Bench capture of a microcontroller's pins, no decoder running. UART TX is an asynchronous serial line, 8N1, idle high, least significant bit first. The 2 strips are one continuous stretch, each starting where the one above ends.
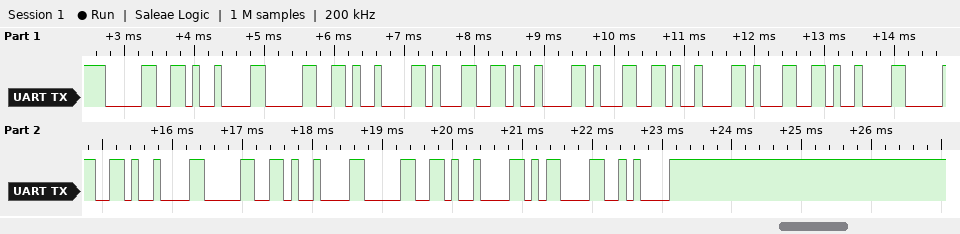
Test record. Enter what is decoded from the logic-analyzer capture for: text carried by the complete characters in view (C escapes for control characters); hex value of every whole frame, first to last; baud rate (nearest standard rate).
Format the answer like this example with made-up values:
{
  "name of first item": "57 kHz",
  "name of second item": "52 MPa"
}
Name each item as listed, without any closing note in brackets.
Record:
{
  "text carried by the complete characters in view": "\"0\\t0\\t1\\t1\\t1\\t0\\t0\\t0\\t\\r\\n\"",
  "hex value of every whole frame, first to last": "30 09 30 09 31 09 31 09 31 09 30 09 30 09 30 09 0D 0A",
  "baud rate": "9600 baud"
}
